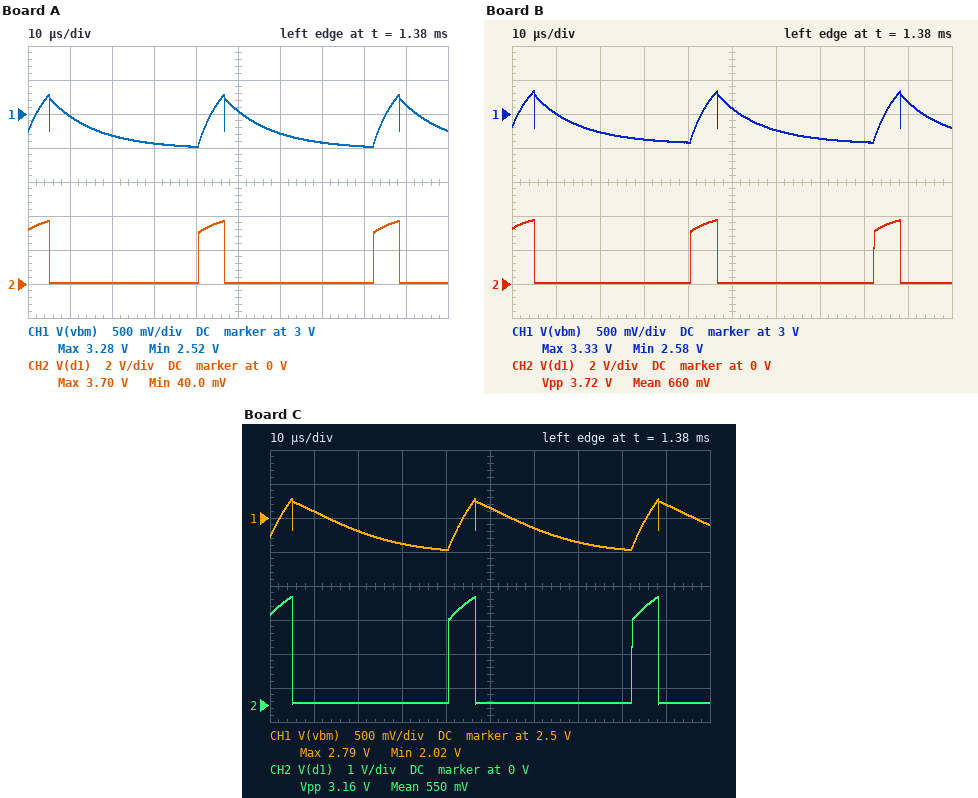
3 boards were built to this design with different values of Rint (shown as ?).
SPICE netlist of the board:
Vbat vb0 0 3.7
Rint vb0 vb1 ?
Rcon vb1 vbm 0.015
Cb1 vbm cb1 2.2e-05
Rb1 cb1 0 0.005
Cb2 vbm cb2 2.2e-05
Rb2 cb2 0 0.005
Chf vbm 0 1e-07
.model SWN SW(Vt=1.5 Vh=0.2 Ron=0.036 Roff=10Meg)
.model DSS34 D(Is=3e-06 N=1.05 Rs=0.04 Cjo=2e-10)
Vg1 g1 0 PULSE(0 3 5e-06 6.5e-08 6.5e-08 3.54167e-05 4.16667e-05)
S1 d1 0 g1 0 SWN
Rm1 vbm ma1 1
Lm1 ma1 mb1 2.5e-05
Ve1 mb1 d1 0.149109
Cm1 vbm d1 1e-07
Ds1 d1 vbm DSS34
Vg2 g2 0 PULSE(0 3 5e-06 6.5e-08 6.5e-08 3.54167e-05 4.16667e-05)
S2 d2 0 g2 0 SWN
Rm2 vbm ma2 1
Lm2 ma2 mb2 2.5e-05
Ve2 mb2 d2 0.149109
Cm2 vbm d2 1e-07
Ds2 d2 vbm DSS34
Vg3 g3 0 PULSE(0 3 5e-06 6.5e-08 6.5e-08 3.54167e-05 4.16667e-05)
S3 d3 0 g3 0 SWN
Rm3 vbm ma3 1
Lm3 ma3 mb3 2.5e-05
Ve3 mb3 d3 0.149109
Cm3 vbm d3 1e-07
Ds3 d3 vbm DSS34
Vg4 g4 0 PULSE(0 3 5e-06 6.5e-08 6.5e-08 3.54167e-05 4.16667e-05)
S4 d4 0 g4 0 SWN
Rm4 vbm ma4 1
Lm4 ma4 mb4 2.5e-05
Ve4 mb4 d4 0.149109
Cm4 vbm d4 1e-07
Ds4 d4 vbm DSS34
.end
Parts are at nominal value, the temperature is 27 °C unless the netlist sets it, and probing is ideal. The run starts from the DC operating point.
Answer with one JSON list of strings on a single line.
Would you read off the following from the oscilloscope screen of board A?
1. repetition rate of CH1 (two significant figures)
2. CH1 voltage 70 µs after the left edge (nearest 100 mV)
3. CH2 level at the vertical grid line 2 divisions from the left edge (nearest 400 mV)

["24 kHz", "2.6 V", "0 V"]
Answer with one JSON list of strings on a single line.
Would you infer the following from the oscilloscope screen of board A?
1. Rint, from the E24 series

["0.12 Ω"]
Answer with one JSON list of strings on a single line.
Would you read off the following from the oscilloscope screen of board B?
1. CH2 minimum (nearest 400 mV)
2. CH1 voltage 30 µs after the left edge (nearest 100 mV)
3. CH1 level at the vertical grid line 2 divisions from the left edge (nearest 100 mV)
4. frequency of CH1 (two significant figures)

["0 V", "2.6 V", "2.7 V", "24 kHz"]
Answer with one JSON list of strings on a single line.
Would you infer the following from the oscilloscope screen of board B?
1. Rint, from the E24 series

["0.11 Ω"]
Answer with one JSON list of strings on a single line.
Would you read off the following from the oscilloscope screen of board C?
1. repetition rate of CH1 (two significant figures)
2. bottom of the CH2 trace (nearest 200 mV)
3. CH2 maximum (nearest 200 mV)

["24 kHz", "0 V", "3.2 V"]
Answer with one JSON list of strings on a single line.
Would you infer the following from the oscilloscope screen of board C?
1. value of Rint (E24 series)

["0.22 Ω"]
